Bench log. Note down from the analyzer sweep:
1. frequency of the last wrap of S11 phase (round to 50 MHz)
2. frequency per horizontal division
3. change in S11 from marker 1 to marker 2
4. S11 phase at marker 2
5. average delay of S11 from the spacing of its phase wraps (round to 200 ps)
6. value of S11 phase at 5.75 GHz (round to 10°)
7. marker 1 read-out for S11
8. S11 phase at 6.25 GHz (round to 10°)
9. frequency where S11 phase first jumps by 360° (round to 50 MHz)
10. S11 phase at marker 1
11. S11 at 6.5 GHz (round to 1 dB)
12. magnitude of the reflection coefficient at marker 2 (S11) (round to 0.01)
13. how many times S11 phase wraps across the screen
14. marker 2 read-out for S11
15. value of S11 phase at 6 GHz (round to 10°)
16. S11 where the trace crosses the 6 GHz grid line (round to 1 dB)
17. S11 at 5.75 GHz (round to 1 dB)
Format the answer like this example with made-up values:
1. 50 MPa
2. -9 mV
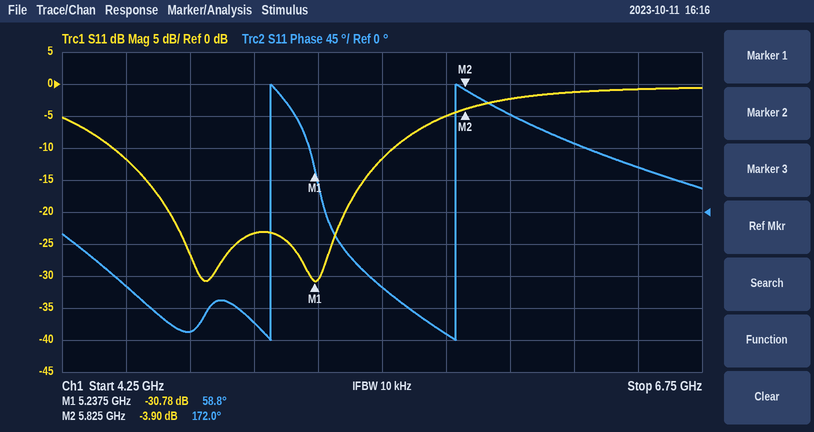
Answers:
1. 5.80 GHz
2. 250 MHz
3. 26.88 dB
4. 172.0°
5. 1.4 ns
6. -170°
7. -30.78 dB
8. 100°
9. 5.05 GHz
10. 58.8°
11. -1 dB
12. 0.64
13. 2
14. -3.90 dB
15. 140°
16. -2 dB
17. -5 dB
